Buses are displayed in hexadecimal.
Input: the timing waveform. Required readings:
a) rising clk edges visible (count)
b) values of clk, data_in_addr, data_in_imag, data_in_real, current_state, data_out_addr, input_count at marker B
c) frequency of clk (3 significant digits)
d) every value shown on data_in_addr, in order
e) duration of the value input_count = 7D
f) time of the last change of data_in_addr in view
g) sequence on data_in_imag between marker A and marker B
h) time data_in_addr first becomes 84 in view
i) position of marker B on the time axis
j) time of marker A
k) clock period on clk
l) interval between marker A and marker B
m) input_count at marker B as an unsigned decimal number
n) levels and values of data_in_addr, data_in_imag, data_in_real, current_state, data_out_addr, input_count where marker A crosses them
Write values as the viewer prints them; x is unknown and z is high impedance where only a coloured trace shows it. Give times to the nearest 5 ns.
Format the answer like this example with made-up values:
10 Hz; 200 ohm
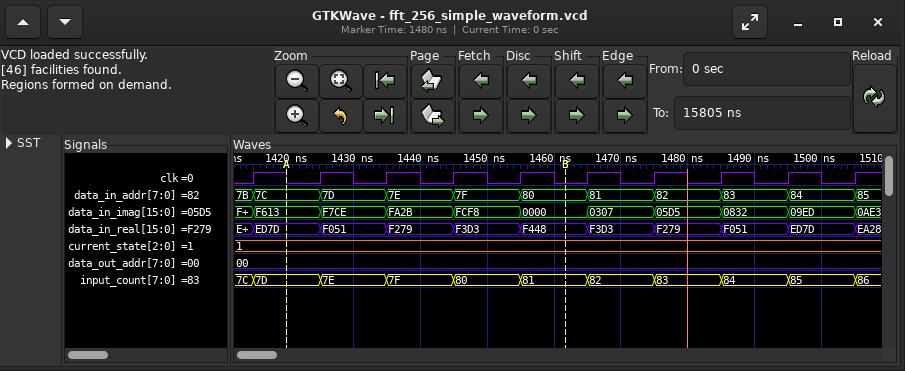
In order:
10; clk=0, data_in_addr=80, data_in_imag=0000, data_in_real=F448, current_state=1, data_out_addr=00, input_count=81; 100 MHz; 7B, 7C, 7D, 7E, 7F, 80, 81, 82, 83, 84, 85; 10 ns; 1505 ns; F613, F7CE, FA2B, FCF8, 0000; 1495 ns; 1460 ns; 1420 ns; 10 ns; 40 ns; 129; data_in_addr=7C, data_in_imag=F613, data_in_real=ED7D, current_state=1, data_out_addr=00, input_count=7D
